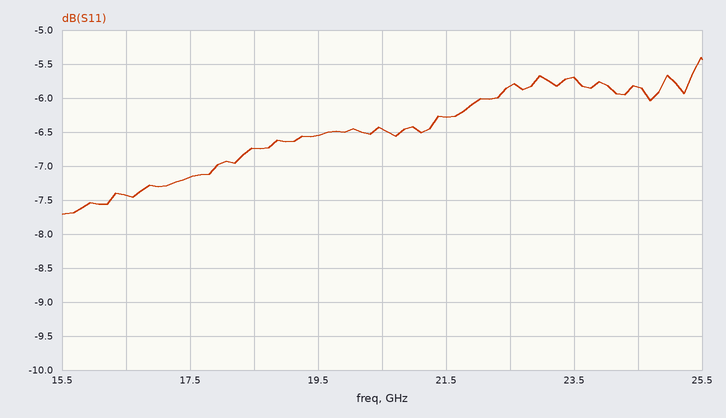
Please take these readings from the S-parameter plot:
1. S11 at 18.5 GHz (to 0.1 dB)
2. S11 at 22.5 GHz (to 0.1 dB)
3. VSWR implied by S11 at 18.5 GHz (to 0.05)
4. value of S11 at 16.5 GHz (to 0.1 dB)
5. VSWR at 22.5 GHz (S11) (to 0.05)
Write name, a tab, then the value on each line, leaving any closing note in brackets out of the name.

S11 at 18.5 GHz	-6.7 dB
S11 at 22.5 GHz	-5.8 dB
VSWR implied by S11 at 18.5 GHz	2.70
value of S11 at 16.5 GHz	-7.4 dB
VSWR at 22.5 GHz (S11)	3.10
